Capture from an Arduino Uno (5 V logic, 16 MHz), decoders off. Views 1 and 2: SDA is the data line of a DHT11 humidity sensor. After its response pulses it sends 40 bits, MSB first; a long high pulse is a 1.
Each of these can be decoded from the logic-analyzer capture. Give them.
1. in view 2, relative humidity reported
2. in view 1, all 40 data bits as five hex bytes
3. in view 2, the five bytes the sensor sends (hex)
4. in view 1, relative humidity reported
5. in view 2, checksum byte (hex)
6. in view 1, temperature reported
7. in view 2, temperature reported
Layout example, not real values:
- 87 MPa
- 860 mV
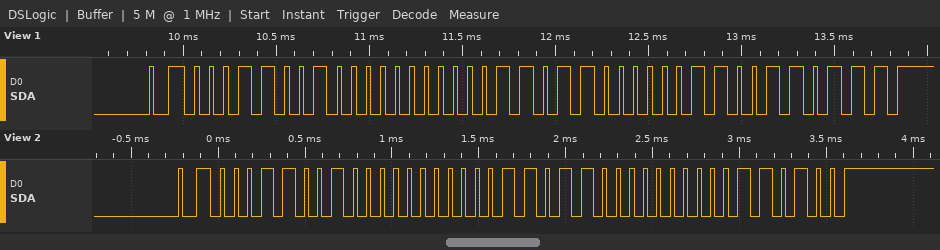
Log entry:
- 25 %
- 19 00 1B 03 37
- 19 00 1B 00 34
- 25 %
- 0x34
- 27.3 °C
- 27.0 °C
